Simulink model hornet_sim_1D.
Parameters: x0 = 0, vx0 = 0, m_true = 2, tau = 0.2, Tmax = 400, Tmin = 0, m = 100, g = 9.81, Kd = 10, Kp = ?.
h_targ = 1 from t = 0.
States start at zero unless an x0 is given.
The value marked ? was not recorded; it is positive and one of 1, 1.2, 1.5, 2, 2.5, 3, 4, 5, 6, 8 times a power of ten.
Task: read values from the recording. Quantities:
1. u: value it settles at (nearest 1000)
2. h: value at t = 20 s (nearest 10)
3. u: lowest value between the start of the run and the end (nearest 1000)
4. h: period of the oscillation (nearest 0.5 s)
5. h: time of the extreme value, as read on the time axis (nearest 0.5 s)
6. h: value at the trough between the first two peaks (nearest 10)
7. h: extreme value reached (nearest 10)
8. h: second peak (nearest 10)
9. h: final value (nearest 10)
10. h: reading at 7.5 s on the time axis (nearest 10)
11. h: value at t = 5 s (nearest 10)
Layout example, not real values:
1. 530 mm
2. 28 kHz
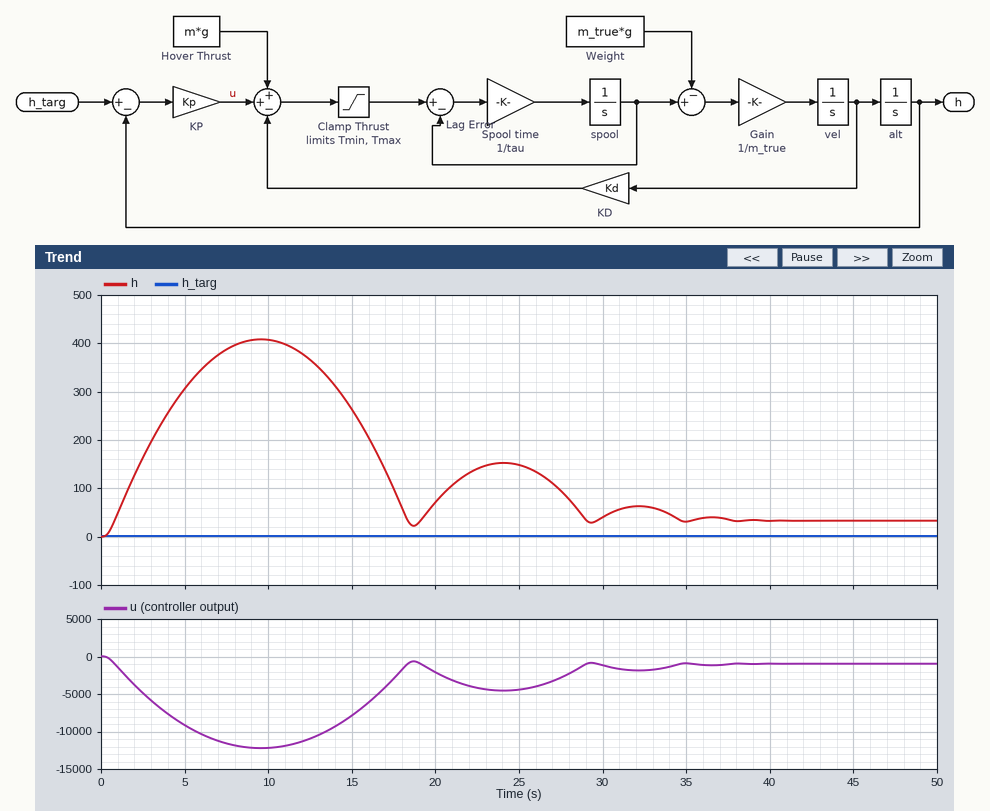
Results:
1. -1000
2. 70
3. -12000
4. 14.5 s
5. 9.5 s
6. 20
7. 410
8. 150
9. 30
10. 390
11. 310
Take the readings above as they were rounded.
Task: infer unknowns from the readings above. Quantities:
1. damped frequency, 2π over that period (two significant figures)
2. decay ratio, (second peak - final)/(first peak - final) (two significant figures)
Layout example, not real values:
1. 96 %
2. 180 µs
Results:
1. 0.43 rad/s
2. 0.32
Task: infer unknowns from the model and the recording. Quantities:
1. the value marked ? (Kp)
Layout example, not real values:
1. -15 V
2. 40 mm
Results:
1. 30
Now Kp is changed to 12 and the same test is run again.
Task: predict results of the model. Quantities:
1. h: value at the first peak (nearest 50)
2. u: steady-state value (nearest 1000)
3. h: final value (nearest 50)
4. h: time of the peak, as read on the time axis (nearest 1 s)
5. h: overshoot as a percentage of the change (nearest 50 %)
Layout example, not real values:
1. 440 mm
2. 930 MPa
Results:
1. 550
2. -1000
3. 100
4. 11 s
5. 550 %
